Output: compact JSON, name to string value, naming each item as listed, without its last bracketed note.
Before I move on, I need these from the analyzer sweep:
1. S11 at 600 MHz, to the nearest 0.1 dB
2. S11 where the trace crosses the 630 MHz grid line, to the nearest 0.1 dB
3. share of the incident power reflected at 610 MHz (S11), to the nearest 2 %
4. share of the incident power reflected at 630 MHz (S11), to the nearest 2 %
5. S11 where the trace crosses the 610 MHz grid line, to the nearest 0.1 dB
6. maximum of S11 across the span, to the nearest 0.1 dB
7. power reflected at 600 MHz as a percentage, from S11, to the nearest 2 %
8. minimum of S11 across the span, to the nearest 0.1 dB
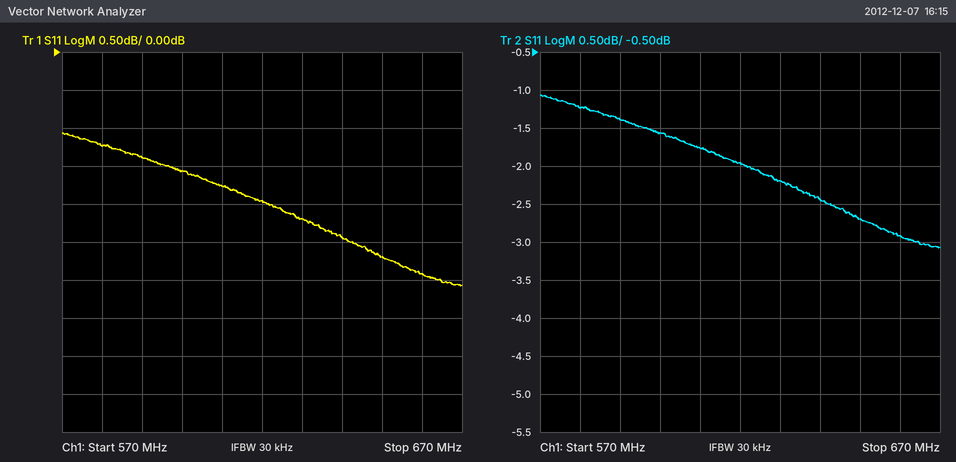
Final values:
{"S11 at 600 MHz, to the nearest 0.1 dB": "-1.6 dB", "S11 where the trace crosses the 630 MHz grid line, to the nearest 0.1 dB": "-2.2 dB", "share of the incident power reflected at 610 MHz (S11), to the nearest 2 %": "66 %", "share of the incident power reflected at 630 MHz (S11), to the nearest 2 %": "60 %", "S11 where the trace crosses the 610 MHz grid line, to the nearest 0.1 dB": "-1.8 dB", "maximum of S11 across the span, to the nearest 0.1 dB": "-1.1 dB", "power reflected at 600 MHz as a percentage, from S11, to the nearest 2 %": "70 %", "minimum of S11 across the span, to the nearest 0.1 dB": "-3.1 dB"}
